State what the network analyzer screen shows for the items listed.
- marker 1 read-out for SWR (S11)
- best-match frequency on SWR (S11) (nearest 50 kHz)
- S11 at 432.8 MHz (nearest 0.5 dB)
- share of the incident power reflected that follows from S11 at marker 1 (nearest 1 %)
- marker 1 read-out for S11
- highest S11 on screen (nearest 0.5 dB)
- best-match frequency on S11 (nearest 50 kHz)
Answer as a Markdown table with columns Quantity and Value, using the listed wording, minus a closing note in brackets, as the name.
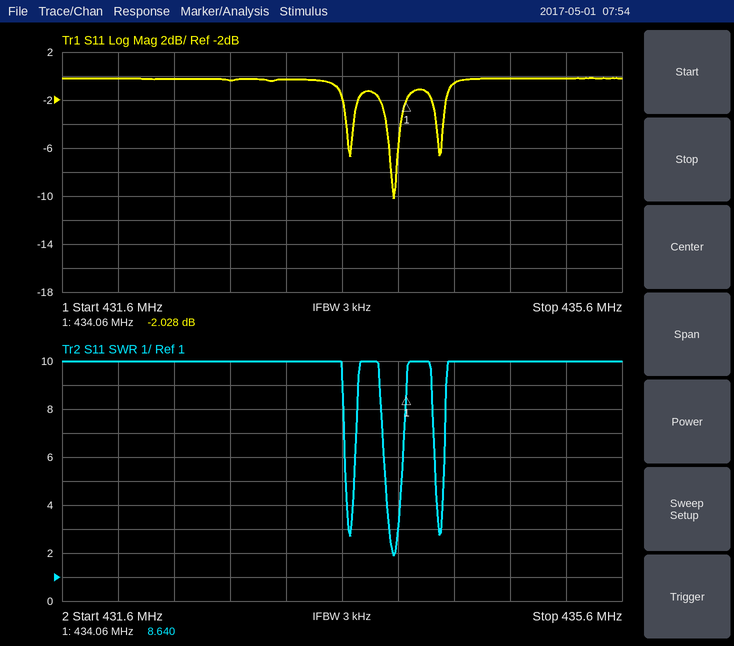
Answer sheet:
| Quantity | Value |
|---|---|
| marker 1 read-out for SWR | 8.640 |
| best-match frequency on SWR (S11) | 433.95 MHz |
| S11 at 432.8 MHz | -0.5 dB |
| share of the incident power reflected that follows from S11 at marker 1 | 63 % |
| marker 1 read-out for S11 | -2.028 dB |
| highest S11 on screen | 0.0 dB |
| best-match frequency on S11 | 433.95 MHz |
